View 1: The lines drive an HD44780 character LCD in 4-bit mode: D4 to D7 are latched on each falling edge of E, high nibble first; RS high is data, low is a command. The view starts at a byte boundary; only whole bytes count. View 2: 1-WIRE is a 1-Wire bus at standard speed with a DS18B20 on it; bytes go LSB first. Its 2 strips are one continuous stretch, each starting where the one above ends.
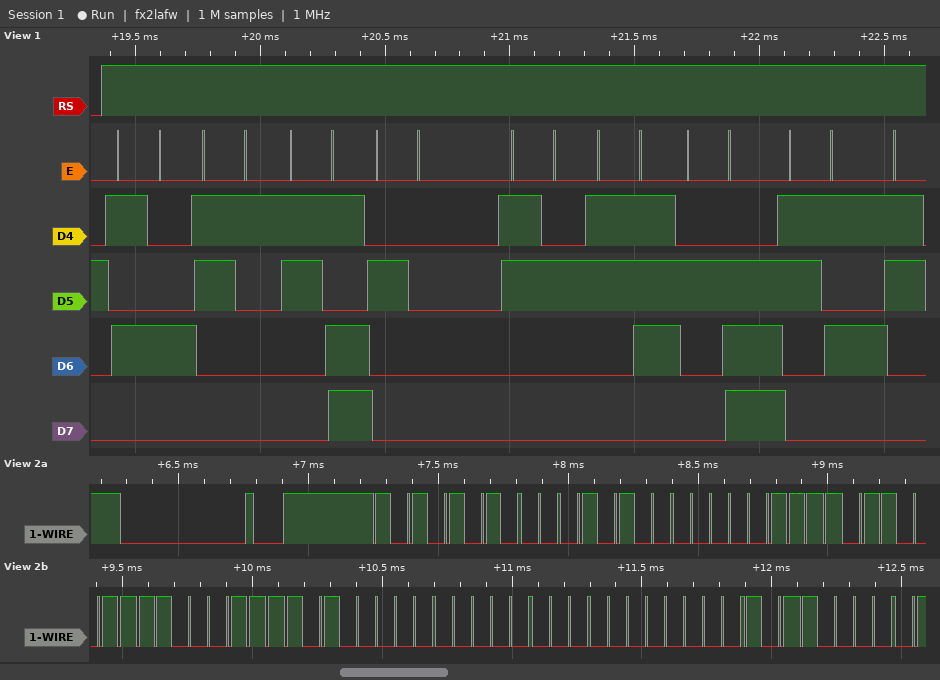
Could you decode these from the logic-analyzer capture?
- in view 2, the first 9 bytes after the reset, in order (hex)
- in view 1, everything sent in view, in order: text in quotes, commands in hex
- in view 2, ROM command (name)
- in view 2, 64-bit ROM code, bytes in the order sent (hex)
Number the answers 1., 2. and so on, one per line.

1. 55 28 E0 CD E3 05 00 00 0D
2. "T1= 27.5"
3. Match ROM
4. 28 E0 CD E3 05 00 00 0D
